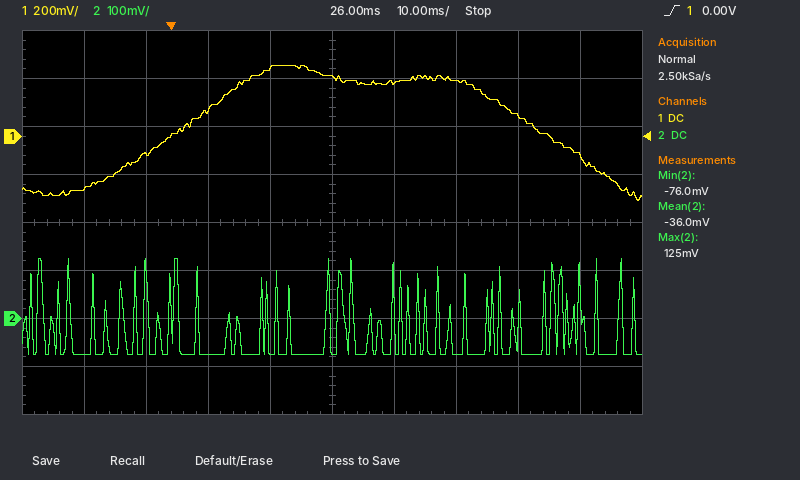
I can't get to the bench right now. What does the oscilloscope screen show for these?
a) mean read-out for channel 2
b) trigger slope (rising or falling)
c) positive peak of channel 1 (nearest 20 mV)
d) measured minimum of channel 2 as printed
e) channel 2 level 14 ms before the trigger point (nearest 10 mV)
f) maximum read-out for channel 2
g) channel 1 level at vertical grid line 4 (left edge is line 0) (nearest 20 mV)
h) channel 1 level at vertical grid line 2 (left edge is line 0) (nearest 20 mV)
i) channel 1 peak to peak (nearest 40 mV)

-36.0 mV
rising
300 mV
-76.0 mV
-80 mV
125 mV
280 mV
-80 mV
560 mV
